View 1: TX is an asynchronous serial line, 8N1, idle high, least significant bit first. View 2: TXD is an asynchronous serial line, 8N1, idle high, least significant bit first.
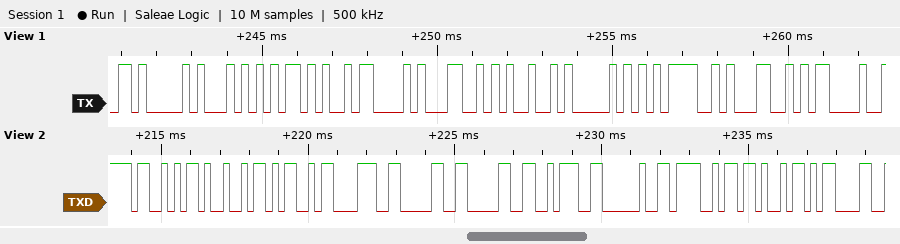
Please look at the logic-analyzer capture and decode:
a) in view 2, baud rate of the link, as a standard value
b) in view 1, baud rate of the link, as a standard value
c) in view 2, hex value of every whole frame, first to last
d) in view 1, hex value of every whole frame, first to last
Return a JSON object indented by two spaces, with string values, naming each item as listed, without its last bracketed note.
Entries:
{
  "in view 2, baud rate of the link, as a standard value": "4800 baud",
  "in view 1, baud rate of the link, as a standard value": "4800 baud",
  "in view 2, hex value of every whole frame, first to last": "53 49 4D 38 30 30 3A 20 4F 4B 0D",
  "in view 1, hex value of every whole frame, first to last": "41 54 2B 43 4C 49 50 3D 31 0D"
}
